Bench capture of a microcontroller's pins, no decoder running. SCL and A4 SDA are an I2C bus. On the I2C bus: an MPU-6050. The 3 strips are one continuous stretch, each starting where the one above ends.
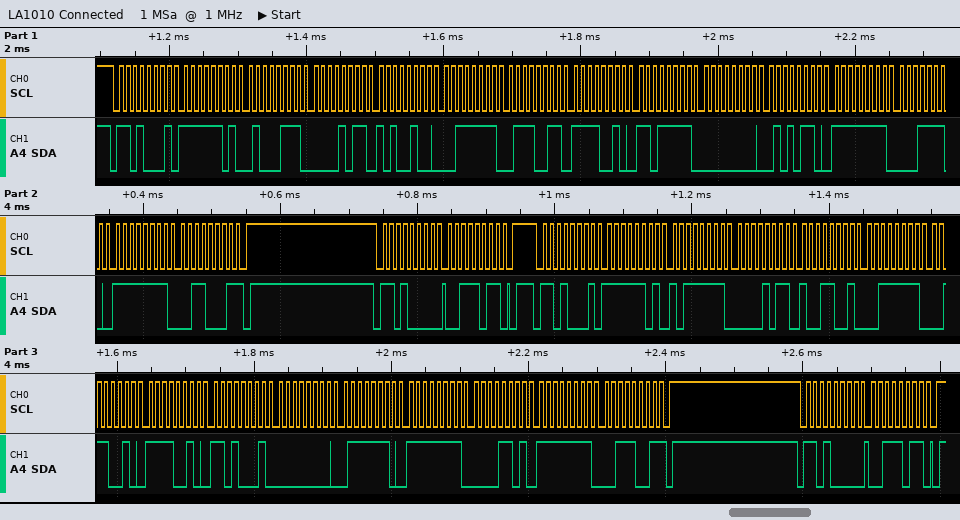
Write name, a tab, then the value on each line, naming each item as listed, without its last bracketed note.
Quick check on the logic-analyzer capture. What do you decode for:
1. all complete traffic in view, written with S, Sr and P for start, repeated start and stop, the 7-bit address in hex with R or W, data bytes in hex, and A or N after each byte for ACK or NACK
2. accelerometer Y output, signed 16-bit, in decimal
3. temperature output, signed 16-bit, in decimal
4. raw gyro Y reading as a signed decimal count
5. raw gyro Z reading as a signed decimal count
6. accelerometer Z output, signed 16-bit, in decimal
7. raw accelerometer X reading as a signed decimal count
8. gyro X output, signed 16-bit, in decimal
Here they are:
all complete traffic in view, written with S, Sr and P for start, repeated start and stop, the 7-bit address in hex with R or W, data bytes in hex, and A or N after each byte for ACK or NACK	S 68R A FD A 47 A 0B A A4 A 3F A 73 A F2 A DF A 00 A 56 A FF A 1E A FF A 31 N P S 68W A 3B A P S 68R A FD A BF A 0B A 99 A 3F A 32 A F2 A D1 A 00 A 7E A FF A 0D A FF A 39 N P S 68W A 3B A P
accelerometer Y output, signed 16-bit, in decimal	2969
temperature output, signed 16-bit, in decimal	-3375
raw gyro Y reading as a signed decimal count	-243
raw gyro Z reading as a signed decimal count	-199
accelerometer Z output, signed 16-bit, in decimal	16178
raw accelerometer X reading as a signed decimal count	-577
gyro X output, signed 16-bit, in decimal	126
